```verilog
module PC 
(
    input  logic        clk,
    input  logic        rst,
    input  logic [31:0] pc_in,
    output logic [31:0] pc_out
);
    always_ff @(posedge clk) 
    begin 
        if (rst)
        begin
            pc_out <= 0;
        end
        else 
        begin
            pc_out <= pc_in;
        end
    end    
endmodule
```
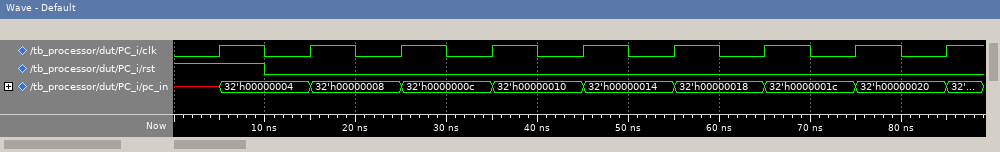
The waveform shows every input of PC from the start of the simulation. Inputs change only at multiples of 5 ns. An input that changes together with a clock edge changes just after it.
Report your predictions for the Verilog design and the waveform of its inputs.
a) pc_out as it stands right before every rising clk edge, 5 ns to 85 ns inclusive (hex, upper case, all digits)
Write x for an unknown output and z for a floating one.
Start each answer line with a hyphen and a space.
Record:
- x, 00000000, 00000004, 00000008, 0000000C, 00000010, 00000014, 00000018, 0000001C
